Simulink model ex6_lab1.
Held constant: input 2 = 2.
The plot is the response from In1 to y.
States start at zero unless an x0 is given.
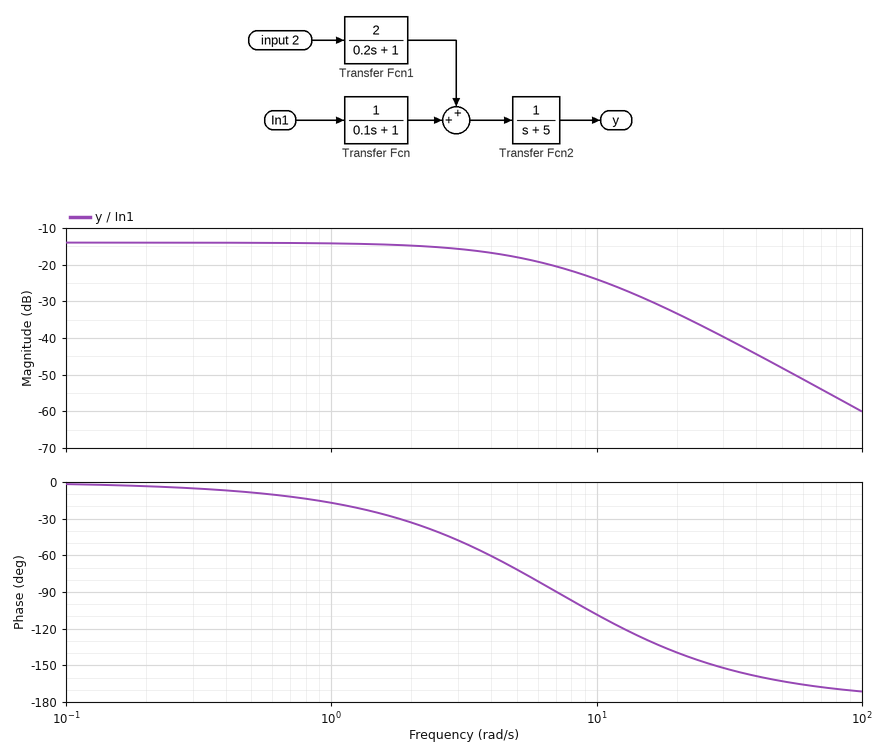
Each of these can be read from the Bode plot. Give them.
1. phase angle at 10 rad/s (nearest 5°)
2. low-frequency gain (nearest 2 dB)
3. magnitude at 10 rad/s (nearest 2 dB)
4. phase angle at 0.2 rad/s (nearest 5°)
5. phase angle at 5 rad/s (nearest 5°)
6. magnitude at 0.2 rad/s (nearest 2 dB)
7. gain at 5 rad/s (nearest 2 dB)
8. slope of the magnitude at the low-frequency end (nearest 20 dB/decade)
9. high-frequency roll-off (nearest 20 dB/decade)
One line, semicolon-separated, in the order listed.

-110°; -14 dB; -24 dB; -5°; -70°; -14 dB; -18 dB; 0 dB/decade; -40 dB/decade
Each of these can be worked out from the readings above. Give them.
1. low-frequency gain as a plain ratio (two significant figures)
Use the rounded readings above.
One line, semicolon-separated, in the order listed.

0.20
